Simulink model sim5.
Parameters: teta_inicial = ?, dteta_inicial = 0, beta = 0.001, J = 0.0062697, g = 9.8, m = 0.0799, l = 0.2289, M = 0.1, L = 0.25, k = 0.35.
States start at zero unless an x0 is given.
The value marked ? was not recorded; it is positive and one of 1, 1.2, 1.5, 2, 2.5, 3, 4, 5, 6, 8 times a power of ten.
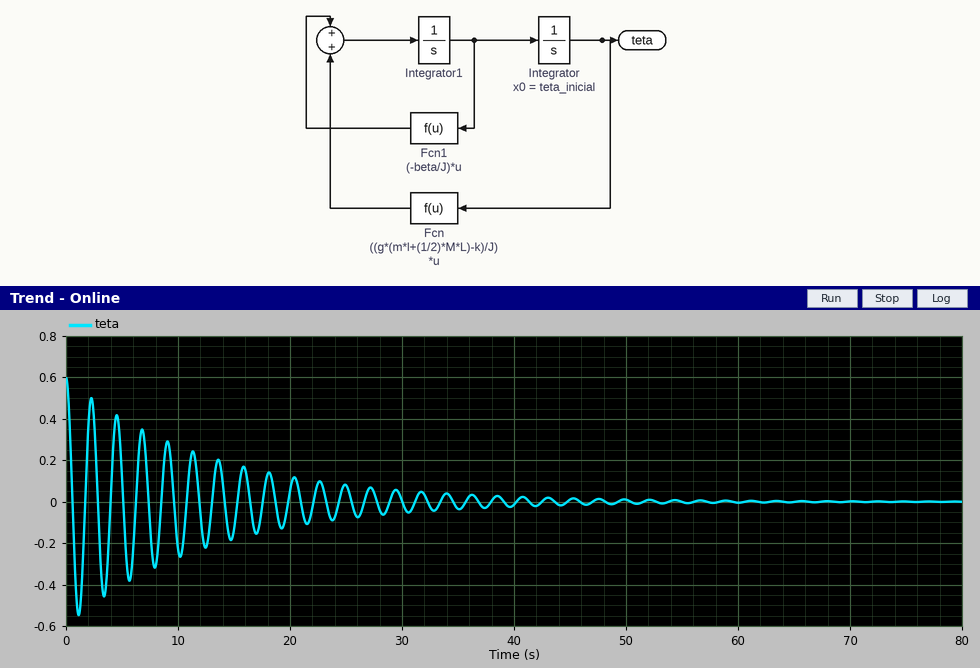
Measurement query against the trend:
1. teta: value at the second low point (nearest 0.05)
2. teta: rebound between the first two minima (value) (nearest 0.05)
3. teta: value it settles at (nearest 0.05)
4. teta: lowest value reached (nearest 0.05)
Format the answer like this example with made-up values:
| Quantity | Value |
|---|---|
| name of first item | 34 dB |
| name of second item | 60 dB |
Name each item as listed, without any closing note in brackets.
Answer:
| Quantity | Value |
|---|---|
| teta: value at the second low point | -0.45 |
| teta: rebound between the first two minima (value) | 0.50 |
| teta: value it settles at | 0.00 |
| teta: lowest value reached | -0.55 |
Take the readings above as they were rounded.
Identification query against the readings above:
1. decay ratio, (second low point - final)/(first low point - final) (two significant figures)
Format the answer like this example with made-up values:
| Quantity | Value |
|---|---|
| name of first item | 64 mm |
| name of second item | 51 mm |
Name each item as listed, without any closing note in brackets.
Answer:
| Quantity | Value |
|---|---|
| decay ratio, (second low point - final)/(first low point - final) | 0.82 |
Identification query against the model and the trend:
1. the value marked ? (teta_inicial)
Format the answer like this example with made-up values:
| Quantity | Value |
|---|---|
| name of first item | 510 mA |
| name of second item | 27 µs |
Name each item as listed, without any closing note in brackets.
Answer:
| Quantity | Value |
|---|---|
| the value marked ? | 0.6 |
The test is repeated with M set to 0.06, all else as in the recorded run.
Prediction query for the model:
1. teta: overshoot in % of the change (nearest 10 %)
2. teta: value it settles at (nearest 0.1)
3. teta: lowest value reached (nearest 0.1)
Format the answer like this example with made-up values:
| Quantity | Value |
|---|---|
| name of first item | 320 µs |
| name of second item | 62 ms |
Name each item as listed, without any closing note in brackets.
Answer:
| Quantity | Value |
|---|---|
| teta: overshoot in % of the change | 90 % |
| teta: value it settles at | 0.0 |
| teta: lowest value reached | -0.6 |
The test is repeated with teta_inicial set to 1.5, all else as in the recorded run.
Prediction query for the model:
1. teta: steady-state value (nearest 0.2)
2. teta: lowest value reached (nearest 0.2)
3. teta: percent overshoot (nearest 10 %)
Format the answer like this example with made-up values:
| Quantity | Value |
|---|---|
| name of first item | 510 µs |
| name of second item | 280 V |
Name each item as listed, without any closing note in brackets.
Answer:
| Quantity | Value |
|---|---|
| teta: steady-state value | 0.0 |
| teta: lowest value reached | -1.4 |
| teta: percent overshoot | 90 % |
